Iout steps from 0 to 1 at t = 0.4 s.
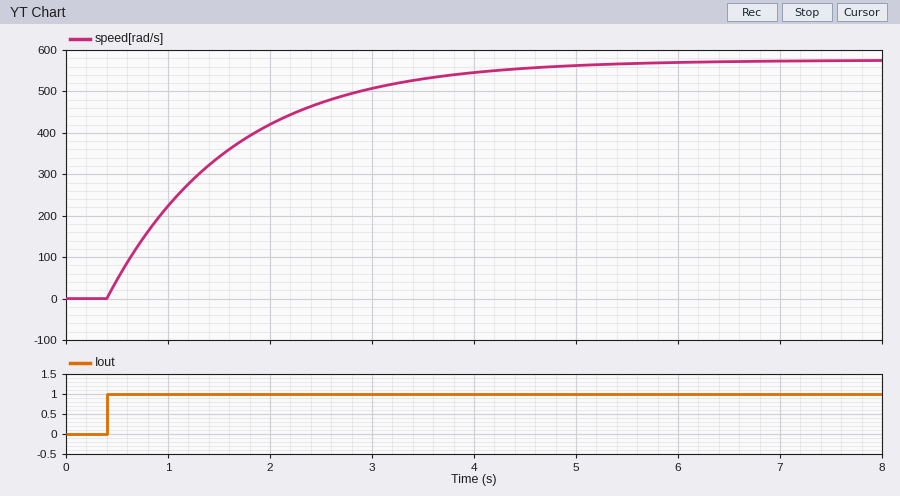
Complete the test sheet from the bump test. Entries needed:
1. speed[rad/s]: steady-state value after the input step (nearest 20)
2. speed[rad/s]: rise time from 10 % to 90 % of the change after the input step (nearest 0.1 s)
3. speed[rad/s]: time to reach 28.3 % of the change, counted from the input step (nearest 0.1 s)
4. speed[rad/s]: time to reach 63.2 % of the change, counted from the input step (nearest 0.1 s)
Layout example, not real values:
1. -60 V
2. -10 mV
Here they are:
1. 580
2. 2.7 s
3. 0.4 s
4. 1.2 s
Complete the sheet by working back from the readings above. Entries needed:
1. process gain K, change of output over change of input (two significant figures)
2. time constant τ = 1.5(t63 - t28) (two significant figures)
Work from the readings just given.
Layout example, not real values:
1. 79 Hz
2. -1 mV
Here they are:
1. 580
2. 1.2 s
